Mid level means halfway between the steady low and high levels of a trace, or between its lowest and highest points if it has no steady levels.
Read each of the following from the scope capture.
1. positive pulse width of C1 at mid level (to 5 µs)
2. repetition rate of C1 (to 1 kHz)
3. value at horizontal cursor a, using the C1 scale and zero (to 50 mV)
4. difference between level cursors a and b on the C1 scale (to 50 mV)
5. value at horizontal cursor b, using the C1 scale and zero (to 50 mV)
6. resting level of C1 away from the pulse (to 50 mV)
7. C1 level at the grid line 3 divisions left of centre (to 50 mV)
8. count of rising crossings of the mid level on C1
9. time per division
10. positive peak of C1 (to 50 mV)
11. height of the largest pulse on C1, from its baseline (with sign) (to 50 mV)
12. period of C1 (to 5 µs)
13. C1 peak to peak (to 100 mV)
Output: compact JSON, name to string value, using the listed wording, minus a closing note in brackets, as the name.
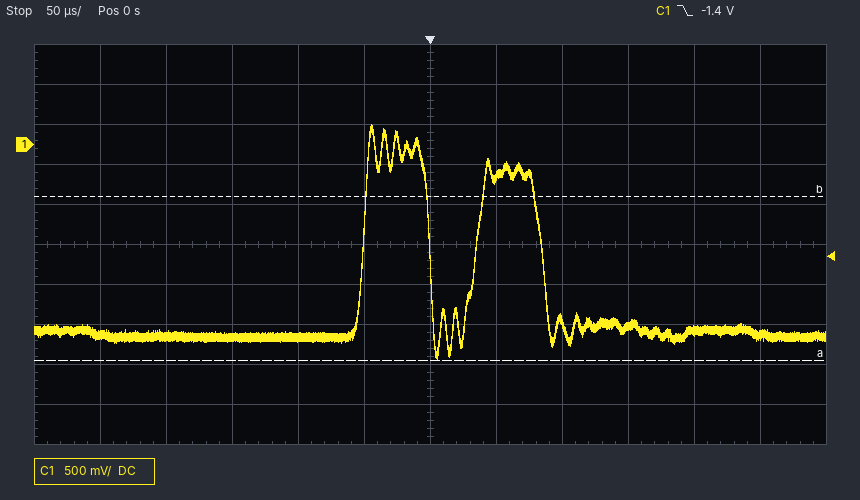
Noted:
{"positive pulse width of C1 at mid level": "50 µs", "repetition rate of C1": "12 kHz", "value at horizontal cursor a, using the C1 scale and zero": "-2.70 V", "difference between level cursors a and b on the C1 scale": "2.05 V", "value at horizontal cursor b, using the C1 scale and zero": "-650 mV", "resting level of C1 away from the pulse": "-2.40 V", "C1 level at the grid line 3 divisions left of centre": "-2.40 V", "count of rising crossings of the mid level on C1": "2", "time per division": "50 µs", "positive peak of C1": "250 mV", "height of the largest pulse on C1, from its baseline (with sign)": "+2.65 V", "period of C1": "85 µs", "C1 peak to peak": "2.90 V"}
